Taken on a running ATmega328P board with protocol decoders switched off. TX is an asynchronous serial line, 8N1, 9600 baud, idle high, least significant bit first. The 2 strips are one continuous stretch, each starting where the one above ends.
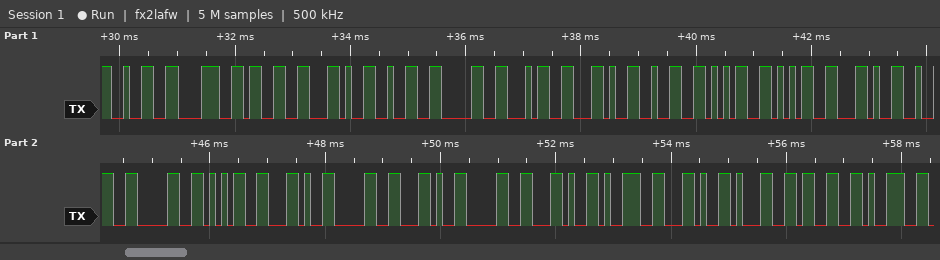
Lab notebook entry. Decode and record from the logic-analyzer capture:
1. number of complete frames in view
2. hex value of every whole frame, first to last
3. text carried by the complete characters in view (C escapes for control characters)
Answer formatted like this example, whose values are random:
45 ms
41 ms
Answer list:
25
0x32 0x38 0x33 0x2C 0x32 0x30 0x34 0x2C 0x32 0x35 0x35 0x2C 0x32 0x30 0x35 0x2C 0x30 0x2C 0x30 0x2C 0x39 0x2C 0x31 0x33 0x39
"283,204,255,205,0,0,9,139"
